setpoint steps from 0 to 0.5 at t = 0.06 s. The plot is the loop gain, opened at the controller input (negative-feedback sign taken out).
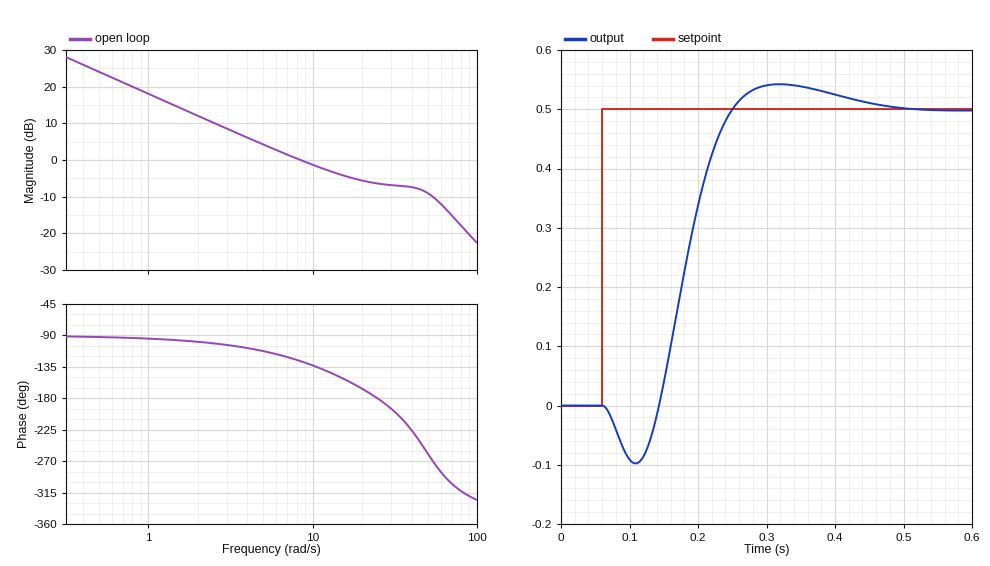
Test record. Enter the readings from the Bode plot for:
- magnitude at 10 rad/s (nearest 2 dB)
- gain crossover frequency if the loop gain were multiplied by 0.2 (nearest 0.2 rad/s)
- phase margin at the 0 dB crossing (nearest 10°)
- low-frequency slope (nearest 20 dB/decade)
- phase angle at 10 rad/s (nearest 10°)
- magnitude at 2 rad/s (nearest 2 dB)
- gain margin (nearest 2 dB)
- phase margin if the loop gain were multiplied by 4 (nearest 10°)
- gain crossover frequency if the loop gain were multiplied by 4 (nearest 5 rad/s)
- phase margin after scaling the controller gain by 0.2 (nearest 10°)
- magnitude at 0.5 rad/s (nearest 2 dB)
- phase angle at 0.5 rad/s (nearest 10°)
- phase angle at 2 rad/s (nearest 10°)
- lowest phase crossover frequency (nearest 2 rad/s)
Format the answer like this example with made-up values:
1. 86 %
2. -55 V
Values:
1. -2 dB
2. 1.6 rad/s
3. 50°
4. -20 dB/decade
5. -130°
6. 12 dB
7. 6 dB
8. -110°
9. 60 rad/s
10. 80°
11. 24 dB
12. -90°
13. -100°
14. 24 rad/s
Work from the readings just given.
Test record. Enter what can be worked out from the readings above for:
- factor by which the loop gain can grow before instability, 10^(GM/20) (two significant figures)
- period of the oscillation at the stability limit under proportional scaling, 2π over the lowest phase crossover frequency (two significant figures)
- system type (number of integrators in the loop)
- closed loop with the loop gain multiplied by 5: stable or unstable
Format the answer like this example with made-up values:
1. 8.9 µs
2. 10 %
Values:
1. 2.0
2. 0.26 s
3. 1
4. unstable
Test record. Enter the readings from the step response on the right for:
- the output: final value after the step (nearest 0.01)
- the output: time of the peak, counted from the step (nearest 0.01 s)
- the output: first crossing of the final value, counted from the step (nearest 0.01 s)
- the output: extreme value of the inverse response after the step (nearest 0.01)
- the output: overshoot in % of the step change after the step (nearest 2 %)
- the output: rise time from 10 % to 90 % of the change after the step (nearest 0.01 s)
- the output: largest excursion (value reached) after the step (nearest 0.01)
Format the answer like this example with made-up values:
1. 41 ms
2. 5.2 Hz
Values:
1. 0.50
2. 0.26 s
3. 0.19 s
4. -0.10
5. 8 %
6. 0.08 s
7. 0.54
